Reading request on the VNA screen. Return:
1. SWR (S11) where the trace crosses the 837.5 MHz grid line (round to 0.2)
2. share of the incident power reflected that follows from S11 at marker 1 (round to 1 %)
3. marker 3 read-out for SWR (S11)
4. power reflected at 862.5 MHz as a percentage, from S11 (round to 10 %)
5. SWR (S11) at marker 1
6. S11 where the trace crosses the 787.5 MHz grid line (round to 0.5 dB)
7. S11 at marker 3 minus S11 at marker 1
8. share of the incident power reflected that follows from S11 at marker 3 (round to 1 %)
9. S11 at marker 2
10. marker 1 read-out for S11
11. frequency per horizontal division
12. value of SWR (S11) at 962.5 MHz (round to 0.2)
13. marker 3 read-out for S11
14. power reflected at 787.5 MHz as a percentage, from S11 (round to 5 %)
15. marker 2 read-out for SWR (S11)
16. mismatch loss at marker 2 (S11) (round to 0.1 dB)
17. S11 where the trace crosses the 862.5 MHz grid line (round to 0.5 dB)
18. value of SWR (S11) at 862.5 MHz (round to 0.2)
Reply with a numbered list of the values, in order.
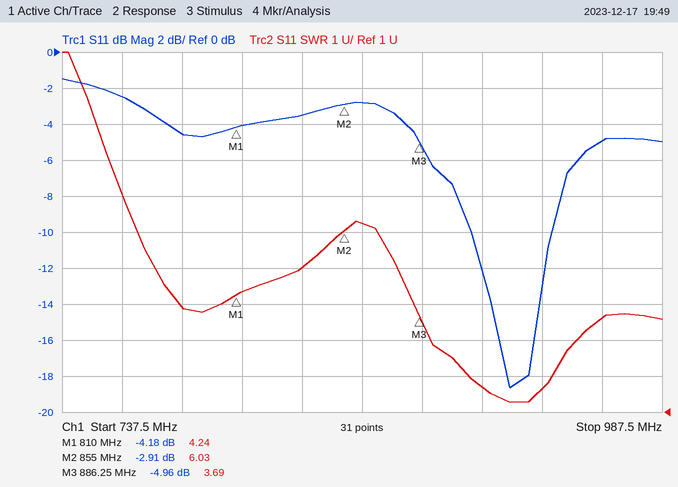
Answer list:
1. 5.0
2. 38 %
3. 3.69
4. 50 %
5. 4.24
6. -4.5 dB
7. -0.78 dB
8. 32 %
9. -2.91 dB
10. -4.18 dB
11. 25 MHz
12. 3.6
13. -4.96 dB
14. 35 %
15. 6.03
16. 3.1 dB
17. -3.0 dB
18. 6.2
